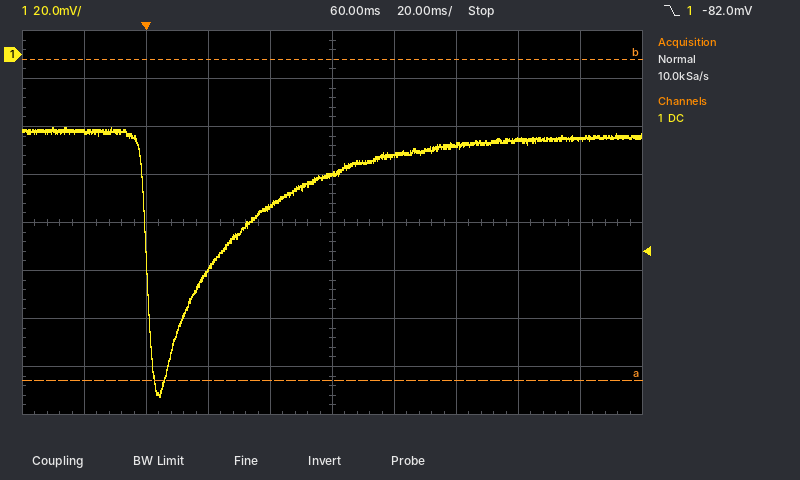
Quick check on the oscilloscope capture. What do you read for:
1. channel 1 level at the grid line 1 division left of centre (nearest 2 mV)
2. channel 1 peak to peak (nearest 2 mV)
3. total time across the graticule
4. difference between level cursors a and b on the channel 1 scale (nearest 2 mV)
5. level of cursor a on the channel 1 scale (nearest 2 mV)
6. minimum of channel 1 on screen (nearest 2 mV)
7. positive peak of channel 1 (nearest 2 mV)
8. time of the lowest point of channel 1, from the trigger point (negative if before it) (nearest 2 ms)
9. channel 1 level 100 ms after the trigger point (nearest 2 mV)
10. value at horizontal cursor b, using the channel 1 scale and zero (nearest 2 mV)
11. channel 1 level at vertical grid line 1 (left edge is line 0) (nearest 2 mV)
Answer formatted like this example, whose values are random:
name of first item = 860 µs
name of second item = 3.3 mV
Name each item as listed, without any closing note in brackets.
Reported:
channel 1 level at the grid line 1 division left of centre = -64 mV
channel 1 peak to peak = 112 mV
total time across the graticule = 200 ms
difference between level cursors a and b on the channel 1 scale = 134 mV
level of cursor a on the channel 1 scale = -136 mV
minimum of channel 1 on screen = -142 mV
positive peak of channel 1 = -30 mV
time of the lowest point of channel 1, from the trigger point (negative if before it) = +4 ms
channel 1 level 100 ms after the trigger point = -38 mV
value at horizontal cursor b, using the channel 1 scale and zero = -2 mV
channel 1 level at vertical grid line 1 (left edge is line 0) = -32 mV
